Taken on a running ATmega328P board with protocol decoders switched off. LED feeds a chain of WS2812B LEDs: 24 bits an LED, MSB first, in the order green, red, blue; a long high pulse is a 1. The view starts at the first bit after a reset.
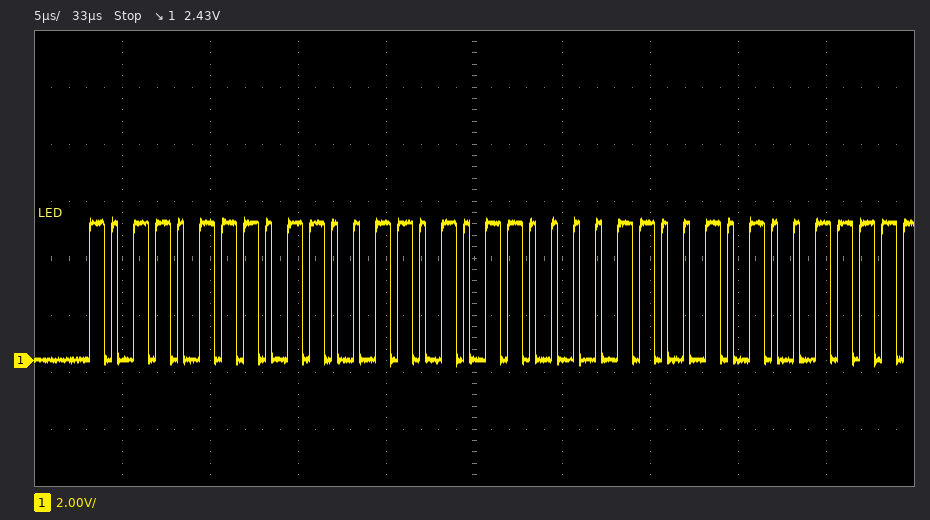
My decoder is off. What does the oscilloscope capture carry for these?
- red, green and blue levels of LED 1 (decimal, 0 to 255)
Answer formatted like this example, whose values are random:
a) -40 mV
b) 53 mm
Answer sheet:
a) 102, 183, 176
